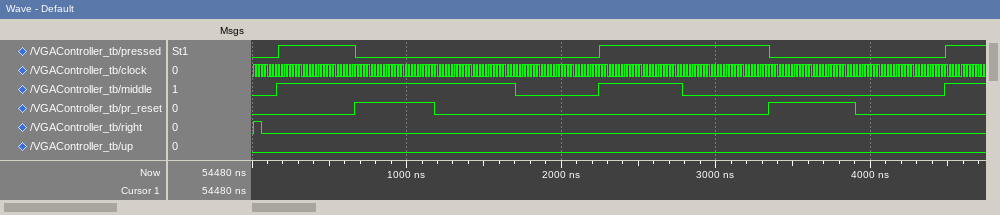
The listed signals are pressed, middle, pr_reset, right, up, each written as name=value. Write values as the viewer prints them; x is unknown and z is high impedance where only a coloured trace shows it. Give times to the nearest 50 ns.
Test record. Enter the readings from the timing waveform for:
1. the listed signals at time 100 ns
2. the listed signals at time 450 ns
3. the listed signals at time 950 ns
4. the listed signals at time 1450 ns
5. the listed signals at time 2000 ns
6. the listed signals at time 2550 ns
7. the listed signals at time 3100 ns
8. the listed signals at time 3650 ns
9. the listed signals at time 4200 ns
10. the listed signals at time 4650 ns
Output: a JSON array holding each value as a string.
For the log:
["pressed=0, middle=0, pr_reset=0, right=0, up=0", "pressed=1, middle=1, pr_reset=0, right=0, up=0", "pressed=0, middle=1, pr_reset=1, right=0, up=0", "pressed=0, middle=1, pr_reset=0, right=0, up=0", "pressed=0, middle=0, pr_reset=0, right=0, up=0", "pressed=1, middle=1, pr_reset=0, right=0, up=0", "pressed=1, middle=0, pr_reset=0, right=0, up=0", "pressed=0, middle=0, pr_reset=1, right=0, up=0", "pressed=0, middle=0, pr_reset=0, right=0, up=0", "pressed=1, middle=1, pr_reset=0, right=0, up=0"]
